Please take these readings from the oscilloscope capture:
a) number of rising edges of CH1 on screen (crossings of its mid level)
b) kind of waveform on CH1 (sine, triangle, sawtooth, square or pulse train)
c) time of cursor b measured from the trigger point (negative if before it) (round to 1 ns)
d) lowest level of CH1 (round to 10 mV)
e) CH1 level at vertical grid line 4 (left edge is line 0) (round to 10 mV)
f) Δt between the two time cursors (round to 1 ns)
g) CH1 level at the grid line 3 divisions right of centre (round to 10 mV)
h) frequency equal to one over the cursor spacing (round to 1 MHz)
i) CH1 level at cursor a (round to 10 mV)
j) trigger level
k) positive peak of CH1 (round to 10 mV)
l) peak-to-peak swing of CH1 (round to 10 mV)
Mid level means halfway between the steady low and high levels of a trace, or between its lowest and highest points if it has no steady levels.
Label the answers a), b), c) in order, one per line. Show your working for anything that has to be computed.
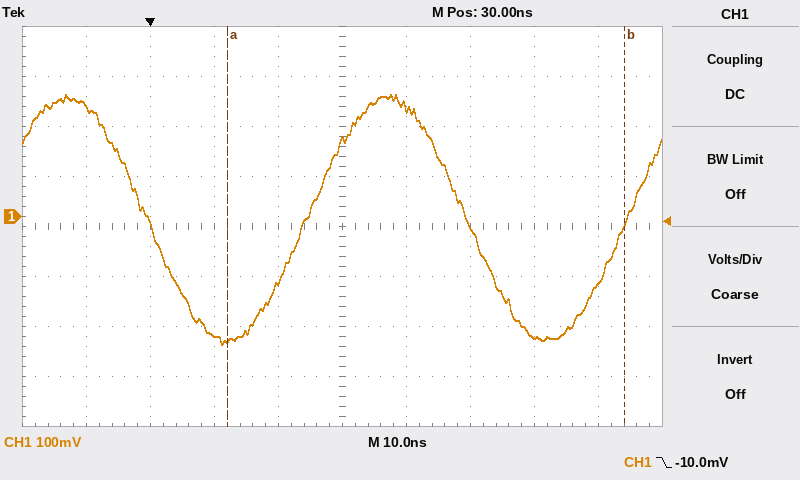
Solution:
a) 2
b) sine
c) +74 ns
d) -260 mV
e) -130 mV
f) 62 ns
g) -240 mV
h) 1 / 62 ns ≈ 16 MHz
i) -250 mV
j) -10.0 mV
k) 240 mV
l) 240 mV − (-260 mV) = 500 mV
